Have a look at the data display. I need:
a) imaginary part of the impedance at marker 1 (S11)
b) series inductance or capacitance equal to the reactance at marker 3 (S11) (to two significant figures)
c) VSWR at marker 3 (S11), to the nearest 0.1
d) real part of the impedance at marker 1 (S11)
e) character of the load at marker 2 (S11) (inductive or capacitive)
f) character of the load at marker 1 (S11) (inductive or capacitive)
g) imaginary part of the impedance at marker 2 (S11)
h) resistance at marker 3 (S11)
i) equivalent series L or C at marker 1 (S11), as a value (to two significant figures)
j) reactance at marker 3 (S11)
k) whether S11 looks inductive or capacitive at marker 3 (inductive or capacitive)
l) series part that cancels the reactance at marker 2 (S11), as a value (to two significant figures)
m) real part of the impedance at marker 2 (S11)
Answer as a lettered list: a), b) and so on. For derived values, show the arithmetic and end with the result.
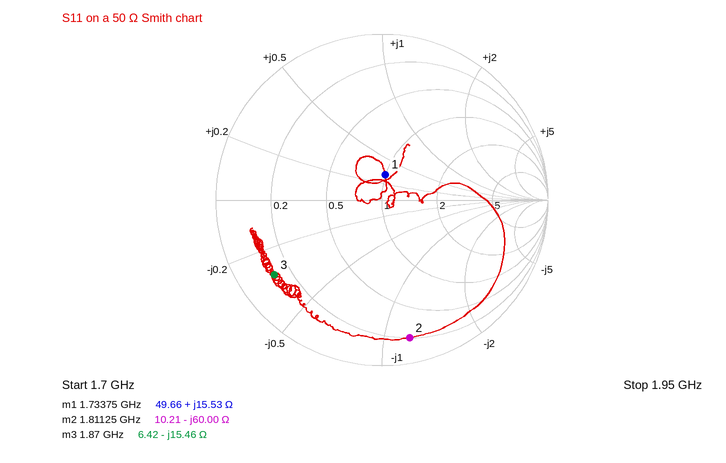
a) +15.53 Ω
b) C = 1/(2π × 1.87 GHz × 15.46 Ω) ≈ 5.5 pF
c) 8.5
d) 49.66 Ω
e) capacitive
f) inductive
g) -60.00 Ω
h) 6.42 Ω
i) L = 15.53 Ω/(2π × 1.73375 GHz) ≈ 1.4 nH
j) -15.46 Ω
k) capacitive
l) L = 60 Ω/(2π × 1.81125 GHz) ≈ 5.3 nH
m) 10.21 Ω
